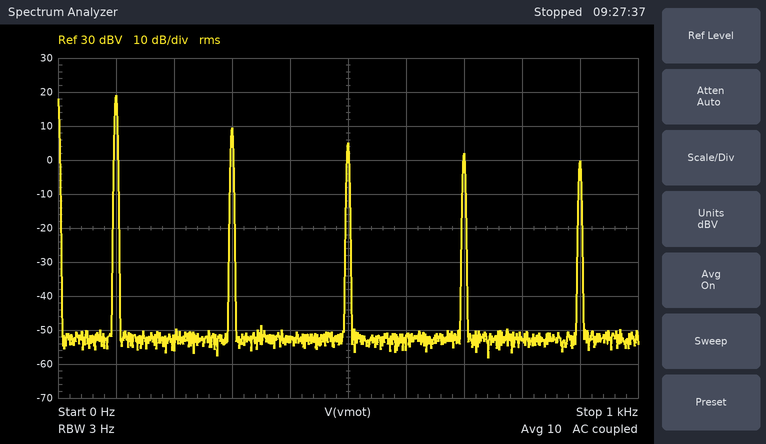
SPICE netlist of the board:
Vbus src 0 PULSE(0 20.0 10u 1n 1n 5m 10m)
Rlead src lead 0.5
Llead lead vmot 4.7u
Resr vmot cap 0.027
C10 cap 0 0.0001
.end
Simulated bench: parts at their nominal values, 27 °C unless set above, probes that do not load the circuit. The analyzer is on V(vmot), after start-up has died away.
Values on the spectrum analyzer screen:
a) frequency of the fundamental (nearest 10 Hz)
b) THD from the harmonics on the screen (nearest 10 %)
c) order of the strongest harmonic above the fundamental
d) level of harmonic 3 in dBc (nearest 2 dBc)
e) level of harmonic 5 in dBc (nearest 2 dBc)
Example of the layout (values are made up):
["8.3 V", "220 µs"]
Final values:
["100 Hz", "40 %", "3", "-10 dBc", "-14 dBc"]
